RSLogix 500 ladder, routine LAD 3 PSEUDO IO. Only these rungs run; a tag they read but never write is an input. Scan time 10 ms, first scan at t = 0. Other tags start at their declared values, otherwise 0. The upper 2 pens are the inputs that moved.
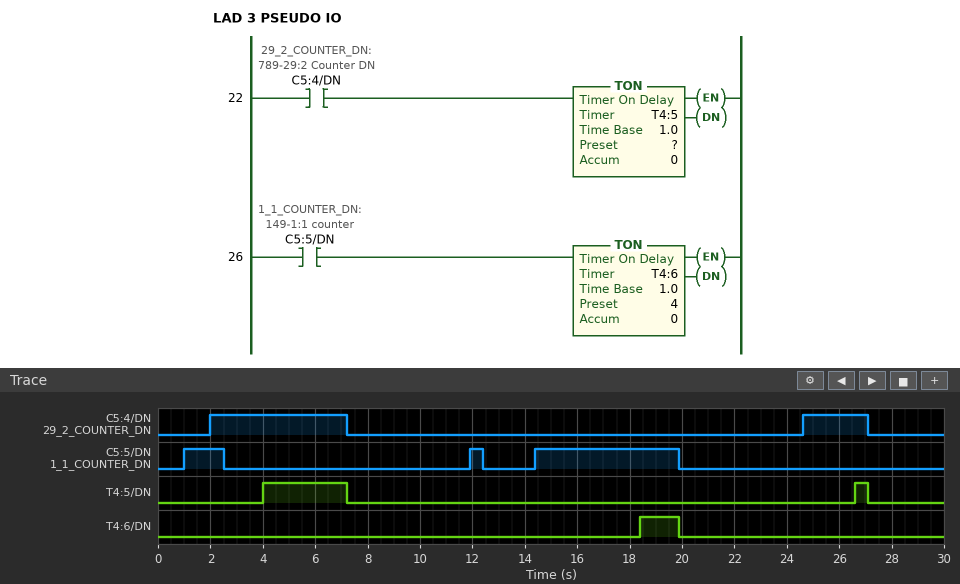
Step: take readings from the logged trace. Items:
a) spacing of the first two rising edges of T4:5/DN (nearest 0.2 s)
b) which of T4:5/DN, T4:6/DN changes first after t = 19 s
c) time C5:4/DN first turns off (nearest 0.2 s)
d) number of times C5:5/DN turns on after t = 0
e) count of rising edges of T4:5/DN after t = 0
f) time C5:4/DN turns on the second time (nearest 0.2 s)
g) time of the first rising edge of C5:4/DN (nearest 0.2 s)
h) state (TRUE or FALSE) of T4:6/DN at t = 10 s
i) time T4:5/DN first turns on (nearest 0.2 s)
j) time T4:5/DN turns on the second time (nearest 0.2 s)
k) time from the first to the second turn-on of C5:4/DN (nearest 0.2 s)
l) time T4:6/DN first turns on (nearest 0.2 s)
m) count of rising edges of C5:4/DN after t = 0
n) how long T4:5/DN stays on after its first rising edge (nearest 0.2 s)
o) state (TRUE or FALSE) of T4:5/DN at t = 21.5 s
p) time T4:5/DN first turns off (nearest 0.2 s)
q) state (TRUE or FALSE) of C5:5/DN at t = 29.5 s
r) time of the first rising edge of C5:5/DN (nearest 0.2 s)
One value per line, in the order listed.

22.6 s
T4:6/DN
7.2 s
3
2
24.6 s
2.0 s
FALSE
4.0 s
26.6 s
22.6 s
18.4 s
2
3.2 s
FALSE
7.2 s
FALSE
1.0 s
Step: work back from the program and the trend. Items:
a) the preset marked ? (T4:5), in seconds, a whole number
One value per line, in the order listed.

2 s
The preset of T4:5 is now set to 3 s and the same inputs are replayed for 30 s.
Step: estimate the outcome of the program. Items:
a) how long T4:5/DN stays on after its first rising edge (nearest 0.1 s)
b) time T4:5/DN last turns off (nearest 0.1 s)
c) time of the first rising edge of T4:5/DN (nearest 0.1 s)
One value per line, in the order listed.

2.2 s
7.2 s
5.0 s
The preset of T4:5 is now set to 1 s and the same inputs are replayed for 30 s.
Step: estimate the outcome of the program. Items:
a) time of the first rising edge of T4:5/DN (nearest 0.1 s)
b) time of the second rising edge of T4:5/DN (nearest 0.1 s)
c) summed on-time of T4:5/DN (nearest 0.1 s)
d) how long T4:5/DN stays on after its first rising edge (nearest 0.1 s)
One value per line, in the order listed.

3.0 s
25.6 s
5.7 s
4.2 s
